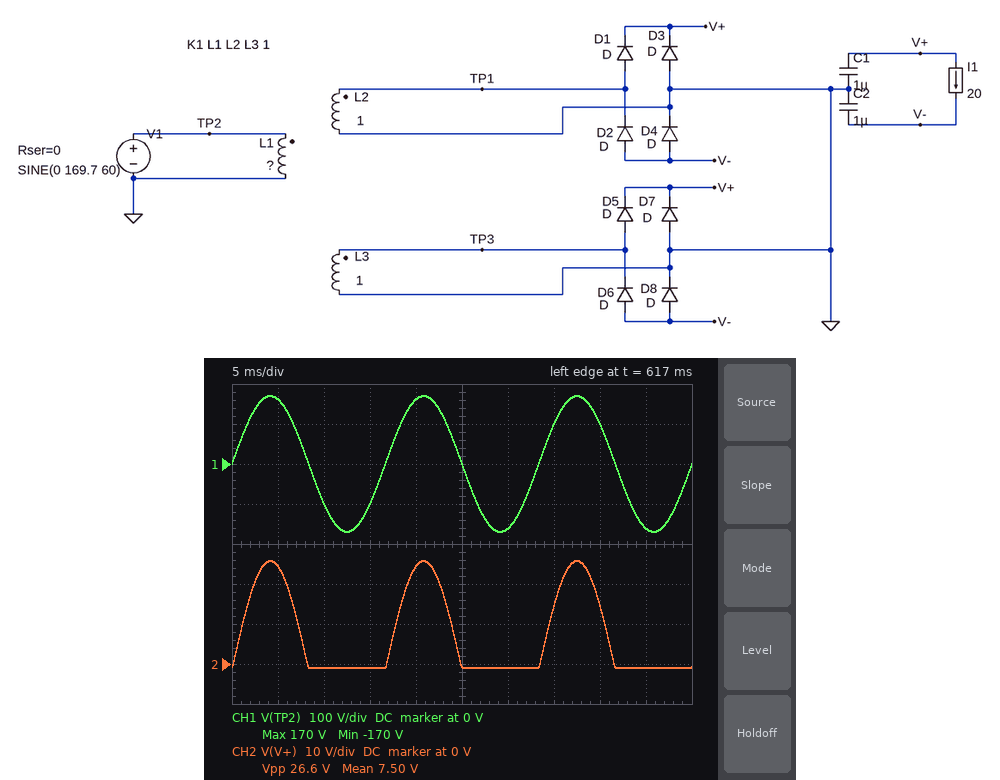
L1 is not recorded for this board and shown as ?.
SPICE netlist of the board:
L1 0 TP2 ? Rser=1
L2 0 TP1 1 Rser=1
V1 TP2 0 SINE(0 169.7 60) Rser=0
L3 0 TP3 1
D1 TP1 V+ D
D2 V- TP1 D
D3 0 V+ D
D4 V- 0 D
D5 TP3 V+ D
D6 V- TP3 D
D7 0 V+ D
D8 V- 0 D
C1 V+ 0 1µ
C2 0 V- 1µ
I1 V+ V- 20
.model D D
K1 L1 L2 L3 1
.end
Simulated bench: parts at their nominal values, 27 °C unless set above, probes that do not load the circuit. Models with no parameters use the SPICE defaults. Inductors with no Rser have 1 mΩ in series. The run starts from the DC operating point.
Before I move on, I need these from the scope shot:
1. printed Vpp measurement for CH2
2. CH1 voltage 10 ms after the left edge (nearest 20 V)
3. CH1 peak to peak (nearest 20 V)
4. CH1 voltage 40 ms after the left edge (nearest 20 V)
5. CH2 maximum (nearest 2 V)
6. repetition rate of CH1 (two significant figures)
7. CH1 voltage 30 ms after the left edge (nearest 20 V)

26.6 V
-100 V
340 V
100 V
26 V
60 Hz
-160 V
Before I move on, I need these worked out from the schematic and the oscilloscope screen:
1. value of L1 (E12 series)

39 H
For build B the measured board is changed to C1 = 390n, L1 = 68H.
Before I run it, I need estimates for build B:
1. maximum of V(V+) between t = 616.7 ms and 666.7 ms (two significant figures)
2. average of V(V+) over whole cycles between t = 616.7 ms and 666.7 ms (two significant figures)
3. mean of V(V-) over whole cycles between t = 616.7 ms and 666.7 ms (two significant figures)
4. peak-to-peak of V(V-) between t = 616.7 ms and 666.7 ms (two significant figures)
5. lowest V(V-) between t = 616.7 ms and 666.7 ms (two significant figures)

19 V
5.5 V
-5.5 V
20 V
-19 V
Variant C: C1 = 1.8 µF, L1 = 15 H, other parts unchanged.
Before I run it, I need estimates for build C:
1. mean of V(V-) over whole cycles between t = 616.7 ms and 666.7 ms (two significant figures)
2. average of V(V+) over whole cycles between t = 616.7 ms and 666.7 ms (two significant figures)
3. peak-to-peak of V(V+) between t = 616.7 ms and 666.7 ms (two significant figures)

-12 V
12 V
42 V
